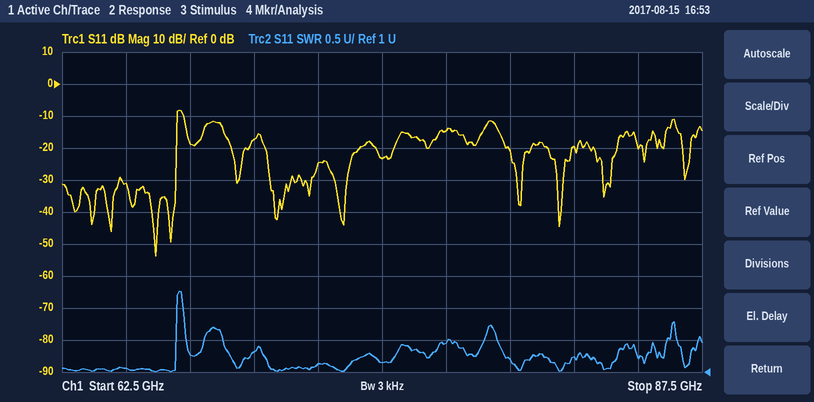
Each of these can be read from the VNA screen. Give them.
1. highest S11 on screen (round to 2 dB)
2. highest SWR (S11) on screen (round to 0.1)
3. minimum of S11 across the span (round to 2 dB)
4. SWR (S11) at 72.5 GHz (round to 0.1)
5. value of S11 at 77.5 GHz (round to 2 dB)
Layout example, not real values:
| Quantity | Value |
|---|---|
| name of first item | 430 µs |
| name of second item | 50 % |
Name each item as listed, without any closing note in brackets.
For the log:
| Quantity | Value |
|---|---|
| highest S11 on screen | -8 dB |
| highest SWR (S11) on screen | 2.3 |
| minimum of S11 across the span | -54 dB |
| SWR (S11) at 72.5 GHz | 1.1 |
| value of S11 at 77.5 GHz | -14 dB |
